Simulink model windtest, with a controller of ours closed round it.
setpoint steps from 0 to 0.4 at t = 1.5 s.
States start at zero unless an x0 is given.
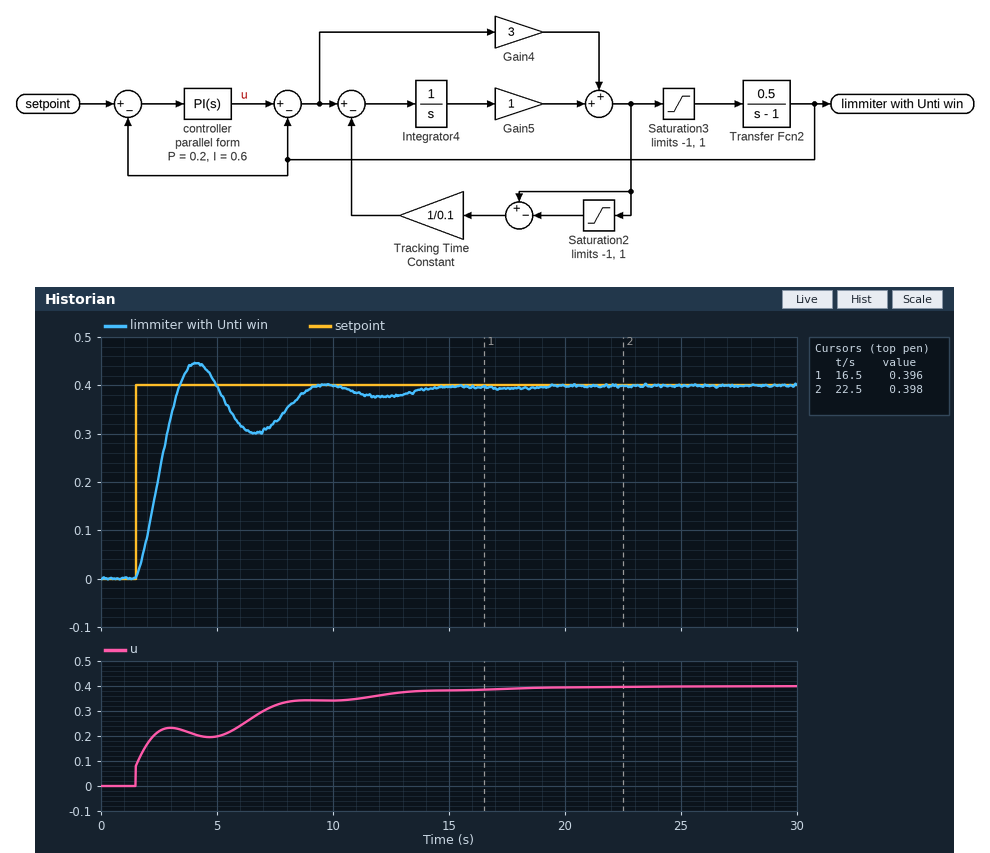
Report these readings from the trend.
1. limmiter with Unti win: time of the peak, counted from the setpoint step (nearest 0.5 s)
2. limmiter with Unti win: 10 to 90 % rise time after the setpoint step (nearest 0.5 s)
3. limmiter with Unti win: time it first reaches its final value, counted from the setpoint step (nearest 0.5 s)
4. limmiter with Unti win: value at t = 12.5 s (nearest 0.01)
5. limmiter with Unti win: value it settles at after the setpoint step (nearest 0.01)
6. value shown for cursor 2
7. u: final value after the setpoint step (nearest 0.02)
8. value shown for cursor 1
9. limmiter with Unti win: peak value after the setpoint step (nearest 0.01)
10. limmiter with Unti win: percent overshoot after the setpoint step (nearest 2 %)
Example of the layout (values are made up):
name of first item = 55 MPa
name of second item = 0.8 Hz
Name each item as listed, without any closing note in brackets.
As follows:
limmiter with Unti win: time of the peak, counted from the setpoint step = 2.5 s
limmiter with Unti win: 10 to 90 % rise time after the setpoint step = 1.5 s
limmiter with Unti win: time it first reaches its final value, counted from the setpoint step = 2.0 s
limmiter with Unti win: value at t = 12.5 s = 0.38
limmiter with Unti win: value it settles at after the setpoint step = 0.40
value shown for cursor 2 = 0.398
u: final value after the setpoint step = 0.40
value shown for cursor 1 = 0.396
limmiter with Unti win: peak value after the setpoint step = 0.45
limmiter with Unti win: percent overshoot after the setpoint step = 12 %
